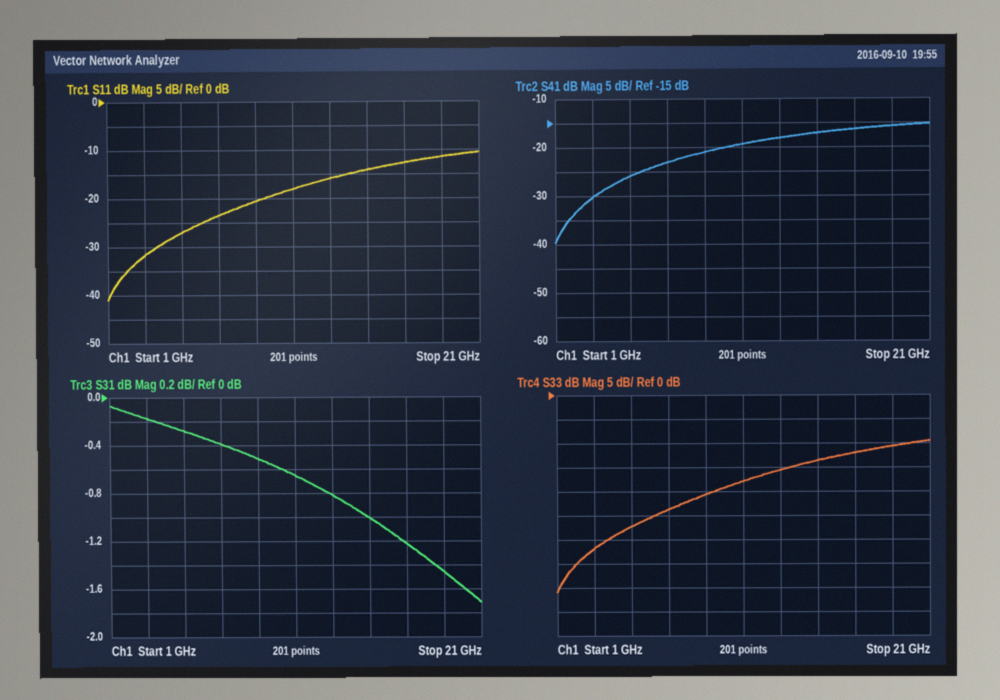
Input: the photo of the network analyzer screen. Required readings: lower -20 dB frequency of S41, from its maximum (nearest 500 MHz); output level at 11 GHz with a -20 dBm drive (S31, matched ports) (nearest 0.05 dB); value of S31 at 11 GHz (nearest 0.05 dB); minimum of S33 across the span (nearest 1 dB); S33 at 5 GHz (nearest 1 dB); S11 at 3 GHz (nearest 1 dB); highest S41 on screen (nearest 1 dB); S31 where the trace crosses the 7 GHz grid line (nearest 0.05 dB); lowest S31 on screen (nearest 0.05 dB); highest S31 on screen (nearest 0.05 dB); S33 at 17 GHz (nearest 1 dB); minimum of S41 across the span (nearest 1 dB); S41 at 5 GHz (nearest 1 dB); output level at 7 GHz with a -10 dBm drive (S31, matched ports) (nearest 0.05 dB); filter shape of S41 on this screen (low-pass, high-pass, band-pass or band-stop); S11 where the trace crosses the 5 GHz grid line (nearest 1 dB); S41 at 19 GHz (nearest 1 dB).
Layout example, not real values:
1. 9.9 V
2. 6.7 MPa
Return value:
1. 1.5 GHz
2. -20.65 dBm
3. -0.65 dB
4. -41 dB
5. -27 dB
6. -32 dB
7. -15 dB
8. -0.40 dB
9. -1.70 dB
10. -0.05 dB
11. -12 dB
12. -40 dB
13. -26 dB
14. -10.40 dBm
15. high-pass
16. -27 dB
17. -16 dB
